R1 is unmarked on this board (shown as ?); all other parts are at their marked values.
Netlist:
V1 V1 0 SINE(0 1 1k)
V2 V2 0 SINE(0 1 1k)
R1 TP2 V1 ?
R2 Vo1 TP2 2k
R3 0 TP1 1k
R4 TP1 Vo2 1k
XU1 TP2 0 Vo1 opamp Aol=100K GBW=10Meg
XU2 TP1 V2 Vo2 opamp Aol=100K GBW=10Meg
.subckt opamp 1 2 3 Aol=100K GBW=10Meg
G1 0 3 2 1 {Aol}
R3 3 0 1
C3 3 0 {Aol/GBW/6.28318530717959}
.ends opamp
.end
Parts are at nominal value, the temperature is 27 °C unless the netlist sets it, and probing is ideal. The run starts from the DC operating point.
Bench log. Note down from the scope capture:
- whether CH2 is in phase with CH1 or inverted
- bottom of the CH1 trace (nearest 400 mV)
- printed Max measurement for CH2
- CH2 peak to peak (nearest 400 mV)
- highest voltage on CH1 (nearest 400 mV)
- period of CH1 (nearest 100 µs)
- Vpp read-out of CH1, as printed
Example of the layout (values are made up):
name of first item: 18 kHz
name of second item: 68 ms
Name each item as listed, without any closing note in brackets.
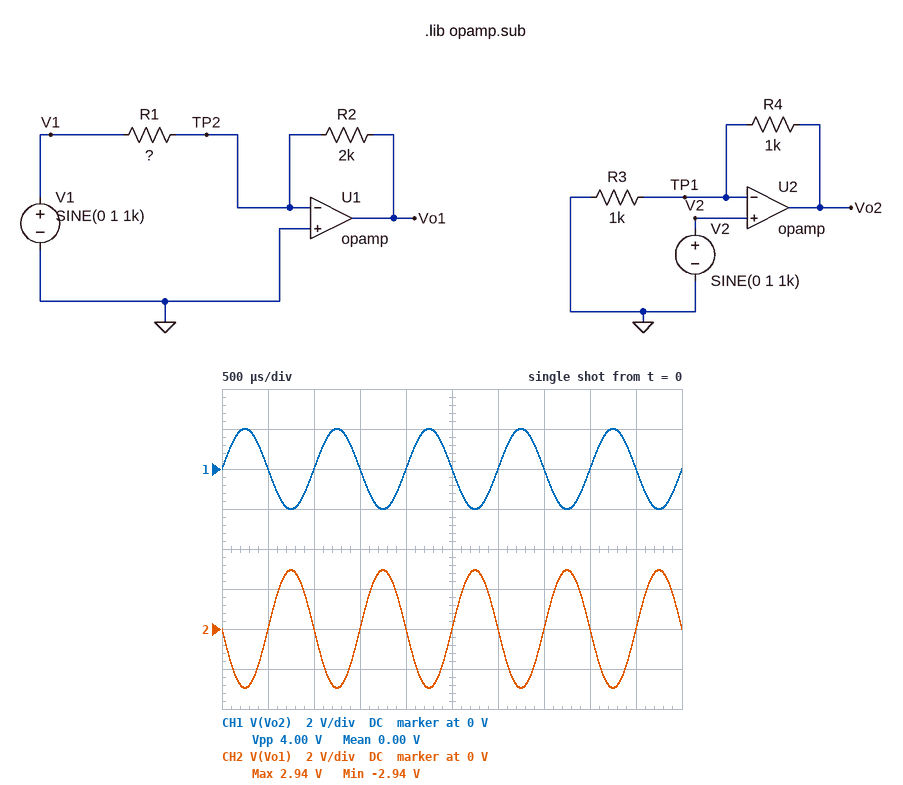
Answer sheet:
whether CH2 is in phase with CH1 or inverted: inverted
bottom of the CH1 trace: -2.0 V
printed Max measurement for CH2: 2.94 V
CH2 peak to peak: 6.0 V
highest voltage on CH1: 2.0 V
period of CH1: 1.0 ms
Vpp read-out of CH1, as printed: 4.00 V
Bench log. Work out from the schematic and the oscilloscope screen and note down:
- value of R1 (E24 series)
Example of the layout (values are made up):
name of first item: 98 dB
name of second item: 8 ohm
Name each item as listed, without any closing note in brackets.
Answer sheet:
value of R1: 680 Ω
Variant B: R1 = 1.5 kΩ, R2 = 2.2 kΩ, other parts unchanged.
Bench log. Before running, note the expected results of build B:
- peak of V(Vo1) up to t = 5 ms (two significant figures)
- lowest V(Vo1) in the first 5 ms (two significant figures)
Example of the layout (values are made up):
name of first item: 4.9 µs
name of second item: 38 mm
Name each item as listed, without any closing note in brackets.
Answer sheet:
peak of V(Vo1) up to t = 5 ms: 1.5 V
lowest V(Vo1) in the first 5 ms: -1.5 V
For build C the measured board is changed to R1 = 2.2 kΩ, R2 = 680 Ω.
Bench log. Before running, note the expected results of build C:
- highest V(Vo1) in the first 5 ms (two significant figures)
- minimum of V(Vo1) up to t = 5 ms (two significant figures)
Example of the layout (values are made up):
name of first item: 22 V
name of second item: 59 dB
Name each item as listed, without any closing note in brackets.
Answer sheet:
highest V(Vo1) in the first 5 ms: 310 mV
minimum of V(Vo1) up to t = 5 ms: -310 mV
